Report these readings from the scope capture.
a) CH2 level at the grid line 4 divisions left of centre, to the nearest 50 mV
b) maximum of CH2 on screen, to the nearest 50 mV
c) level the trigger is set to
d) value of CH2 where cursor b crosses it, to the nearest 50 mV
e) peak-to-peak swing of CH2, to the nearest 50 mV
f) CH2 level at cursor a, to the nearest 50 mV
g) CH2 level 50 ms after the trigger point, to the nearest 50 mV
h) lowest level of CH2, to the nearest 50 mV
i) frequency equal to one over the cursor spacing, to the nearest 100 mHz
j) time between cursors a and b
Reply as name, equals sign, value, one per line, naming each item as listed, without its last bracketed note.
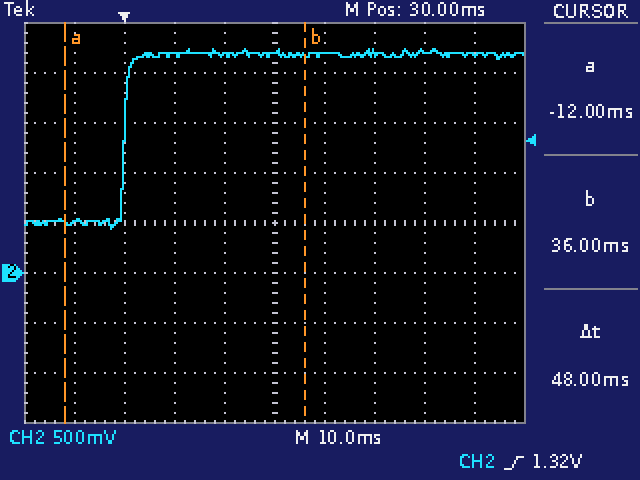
CH2 level at the grid line 4 divisions left of centre, to the nearest 50 mV = 500 mV
maximum of CH2 on screen, to the nearest 50 mV = 2.25 V
level the trigger is set to = 1.32 V
value of CH2 where cursor b crosses it, to the nearest 50 mV = 2.20 V
peak-to-peak swing of CH2, to the nearest 50 mV = 1.80 V
CH2 level at cursor a, to the nearest 50 mV = 500 mV
CH2 level 50 ms after the trigger point, to the nearest 50 mV = 2.20 V
lowest level of CH2, to the nearest 50 mV = 450 mV
frequency equal to one over the cursor spacing, to the nearest 100 mHz = 20.8 Hz
time between cursors a and b = 48 ms
